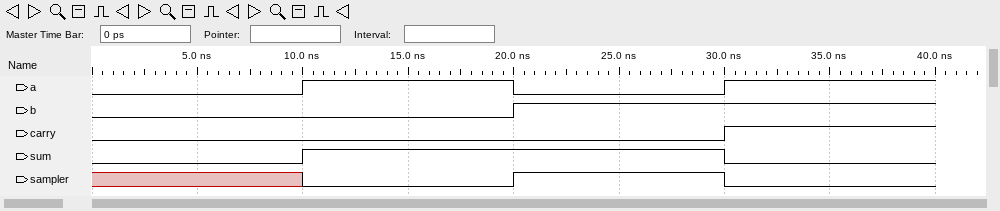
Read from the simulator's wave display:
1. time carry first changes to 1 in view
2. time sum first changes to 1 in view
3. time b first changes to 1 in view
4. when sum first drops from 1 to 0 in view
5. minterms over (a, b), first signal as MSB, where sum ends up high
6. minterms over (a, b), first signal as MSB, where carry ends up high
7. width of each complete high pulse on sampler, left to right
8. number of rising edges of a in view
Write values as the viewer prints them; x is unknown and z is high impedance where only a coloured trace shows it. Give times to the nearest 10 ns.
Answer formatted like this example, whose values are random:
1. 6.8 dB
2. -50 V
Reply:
1. 30 ns
2. 10 ns
3. 20 ns
4. 30 ns
5. 1, 2
6. 3
7. 10 ns
8. 2
